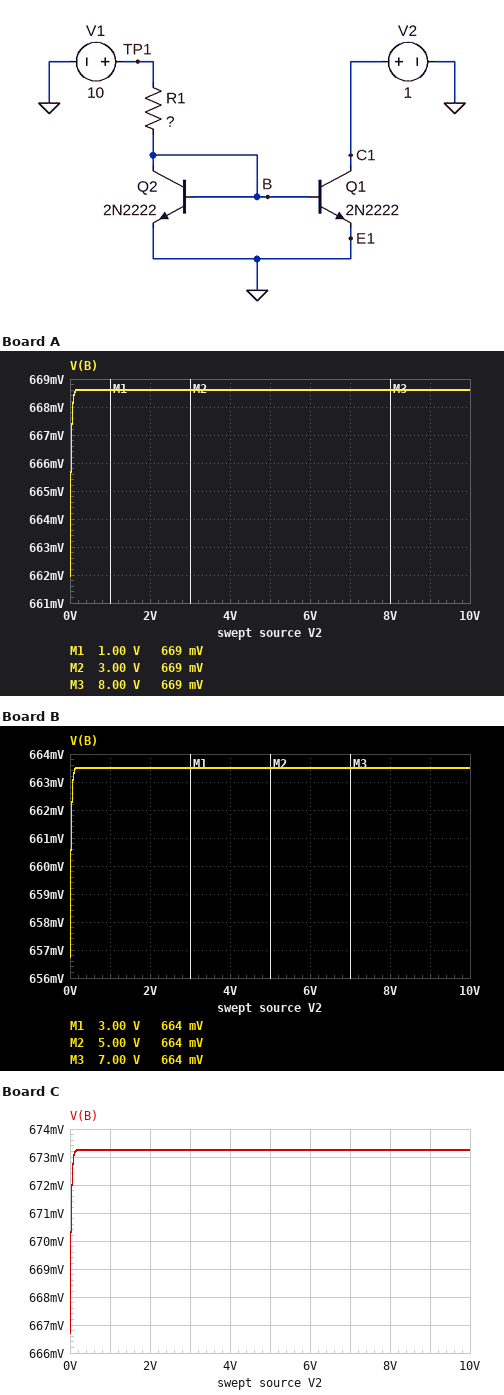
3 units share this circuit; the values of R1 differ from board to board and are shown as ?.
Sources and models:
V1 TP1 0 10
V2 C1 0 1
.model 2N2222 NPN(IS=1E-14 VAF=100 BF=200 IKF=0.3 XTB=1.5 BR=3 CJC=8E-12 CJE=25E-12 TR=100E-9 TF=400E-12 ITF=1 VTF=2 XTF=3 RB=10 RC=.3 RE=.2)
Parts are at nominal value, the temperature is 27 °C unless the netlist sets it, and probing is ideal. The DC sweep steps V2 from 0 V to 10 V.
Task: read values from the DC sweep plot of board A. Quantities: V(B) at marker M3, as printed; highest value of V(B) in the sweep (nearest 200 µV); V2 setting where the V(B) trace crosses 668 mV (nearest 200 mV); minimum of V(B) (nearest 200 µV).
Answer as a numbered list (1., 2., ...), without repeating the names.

1. 669 mV
2. 668.6 mV
3. 0 V
4. 662.0 mV
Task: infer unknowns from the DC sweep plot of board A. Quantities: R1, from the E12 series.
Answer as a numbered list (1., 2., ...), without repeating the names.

1. 5.6 kΩ
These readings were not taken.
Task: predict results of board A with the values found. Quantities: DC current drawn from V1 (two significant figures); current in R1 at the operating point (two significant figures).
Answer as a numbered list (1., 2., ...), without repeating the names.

1. 1.7 mA
2. 1.7 mA
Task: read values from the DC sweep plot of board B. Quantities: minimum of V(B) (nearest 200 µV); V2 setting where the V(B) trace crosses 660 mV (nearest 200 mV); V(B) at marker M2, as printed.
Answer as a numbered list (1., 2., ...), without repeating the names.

1. 656.8 mV
2. 0 V
3. 664 mV
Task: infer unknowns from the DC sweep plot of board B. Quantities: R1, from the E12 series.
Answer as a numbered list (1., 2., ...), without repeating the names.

1. 6.8 kΩ
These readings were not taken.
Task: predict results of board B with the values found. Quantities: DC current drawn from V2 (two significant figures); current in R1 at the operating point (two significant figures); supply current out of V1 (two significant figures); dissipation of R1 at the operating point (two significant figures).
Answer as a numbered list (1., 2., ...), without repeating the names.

1. 1.4 mA
2. 1.4 mA
3. 1.4 mA
4. 13 mW
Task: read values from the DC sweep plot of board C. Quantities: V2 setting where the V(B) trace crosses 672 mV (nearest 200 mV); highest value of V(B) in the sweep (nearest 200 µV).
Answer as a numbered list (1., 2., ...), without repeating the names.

1. 0 V
2. 673.2 mV
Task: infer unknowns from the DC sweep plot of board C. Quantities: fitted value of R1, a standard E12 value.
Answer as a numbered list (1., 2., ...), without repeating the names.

1. 4.7 kΩ
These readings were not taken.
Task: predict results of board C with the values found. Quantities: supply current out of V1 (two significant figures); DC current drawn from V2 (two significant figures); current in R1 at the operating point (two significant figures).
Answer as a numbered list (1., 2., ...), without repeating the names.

1. 2.0 mA
2. 2.0 mA
3. 2.0 mA
